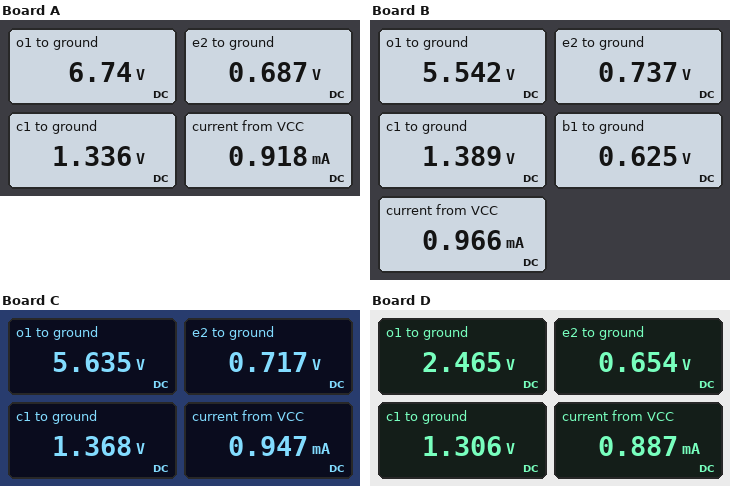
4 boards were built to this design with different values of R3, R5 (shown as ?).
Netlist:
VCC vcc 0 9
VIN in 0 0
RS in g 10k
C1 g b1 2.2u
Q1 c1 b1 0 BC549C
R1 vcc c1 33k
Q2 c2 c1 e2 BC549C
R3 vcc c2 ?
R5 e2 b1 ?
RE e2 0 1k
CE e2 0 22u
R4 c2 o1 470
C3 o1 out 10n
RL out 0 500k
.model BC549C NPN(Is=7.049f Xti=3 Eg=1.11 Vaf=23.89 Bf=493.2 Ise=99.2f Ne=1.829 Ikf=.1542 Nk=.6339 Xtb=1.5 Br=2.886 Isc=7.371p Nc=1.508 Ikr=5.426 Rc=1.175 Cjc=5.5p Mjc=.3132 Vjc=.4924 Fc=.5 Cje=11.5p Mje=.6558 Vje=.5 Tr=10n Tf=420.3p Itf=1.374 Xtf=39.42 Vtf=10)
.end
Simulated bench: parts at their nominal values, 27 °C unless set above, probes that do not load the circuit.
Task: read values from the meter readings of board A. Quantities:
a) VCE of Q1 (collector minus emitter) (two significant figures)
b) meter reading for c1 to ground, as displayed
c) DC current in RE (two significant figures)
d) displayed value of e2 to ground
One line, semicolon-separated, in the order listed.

1.3 V; 1.336 V; 690 µA; 0.687 V
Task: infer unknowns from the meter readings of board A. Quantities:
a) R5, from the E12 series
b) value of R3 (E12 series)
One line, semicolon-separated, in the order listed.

120 kΩ; 3.3 kΩ
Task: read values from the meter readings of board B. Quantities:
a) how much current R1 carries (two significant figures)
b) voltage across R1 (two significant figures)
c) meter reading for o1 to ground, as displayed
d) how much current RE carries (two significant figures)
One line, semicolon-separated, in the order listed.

230 µA; 7.6 V; 5.542 V; 740 µA
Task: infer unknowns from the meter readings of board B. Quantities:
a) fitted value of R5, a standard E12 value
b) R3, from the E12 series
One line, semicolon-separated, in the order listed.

220 kΩ; 4.7 kΩ
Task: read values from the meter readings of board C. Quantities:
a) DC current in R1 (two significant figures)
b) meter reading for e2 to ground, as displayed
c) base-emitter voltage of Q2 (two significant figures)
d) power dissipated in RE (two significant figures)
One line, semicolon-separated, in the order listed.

230 µA; 0.717 V; 650 mV; 510 µW
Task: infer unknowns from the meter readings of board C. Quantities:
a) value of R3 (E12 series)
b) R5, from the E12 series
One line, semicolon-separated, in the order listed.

4.7 kΩ; 180 kΩ
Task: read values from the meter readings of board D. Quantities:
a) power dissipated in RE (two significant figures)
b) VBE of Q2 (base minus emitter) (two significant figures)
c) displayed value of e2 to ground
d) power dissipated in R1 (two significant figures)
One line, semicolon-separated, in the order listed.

430 µW; 650 mV; 0.654 V; 1.8 mW
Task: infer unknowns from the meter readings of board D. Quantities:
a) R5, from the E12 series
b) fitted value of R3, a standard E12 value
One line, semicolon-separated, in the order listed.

56 kΩ; 10 kΩ
